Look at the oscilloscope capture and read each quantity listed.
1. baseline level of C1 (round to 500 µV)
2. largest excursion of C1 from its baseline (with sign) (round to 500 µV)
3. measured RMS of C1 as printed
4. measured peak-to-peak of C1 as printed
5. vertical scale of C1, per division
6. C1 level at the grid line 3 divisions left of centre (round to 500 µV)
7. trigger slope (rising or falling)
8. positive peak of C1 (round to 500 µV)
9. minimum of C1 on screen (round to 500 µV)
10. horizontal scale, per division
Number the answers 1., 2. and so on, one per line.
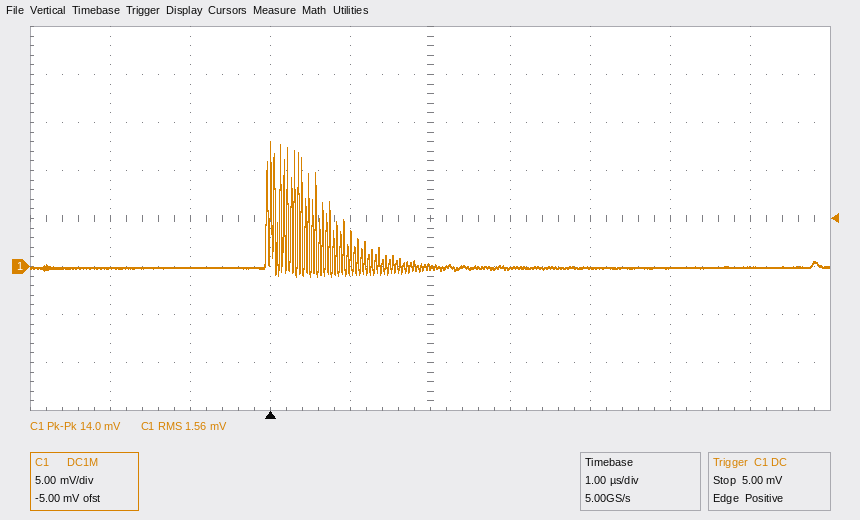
1. 0.0 mV
2. +13.0 mV
3. 1.56 mV
4. 14.0 mV
5. 5 mV
6. 0.0 mV
7. rising
8. 13.0 mV
9. -1.0 mV
10. 1 µs
